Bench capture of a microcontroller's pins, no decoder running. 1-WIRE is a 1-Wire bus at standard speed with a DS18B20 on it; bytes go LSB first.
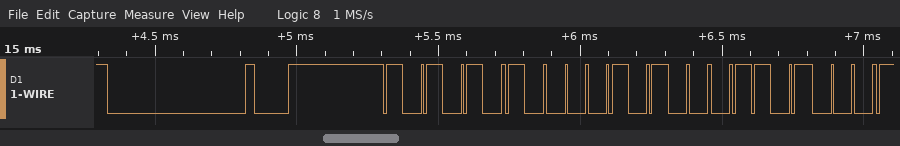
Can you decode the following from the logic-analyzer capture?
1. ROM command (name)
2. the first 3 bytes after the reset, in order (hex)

Match ROM
55 28 16
